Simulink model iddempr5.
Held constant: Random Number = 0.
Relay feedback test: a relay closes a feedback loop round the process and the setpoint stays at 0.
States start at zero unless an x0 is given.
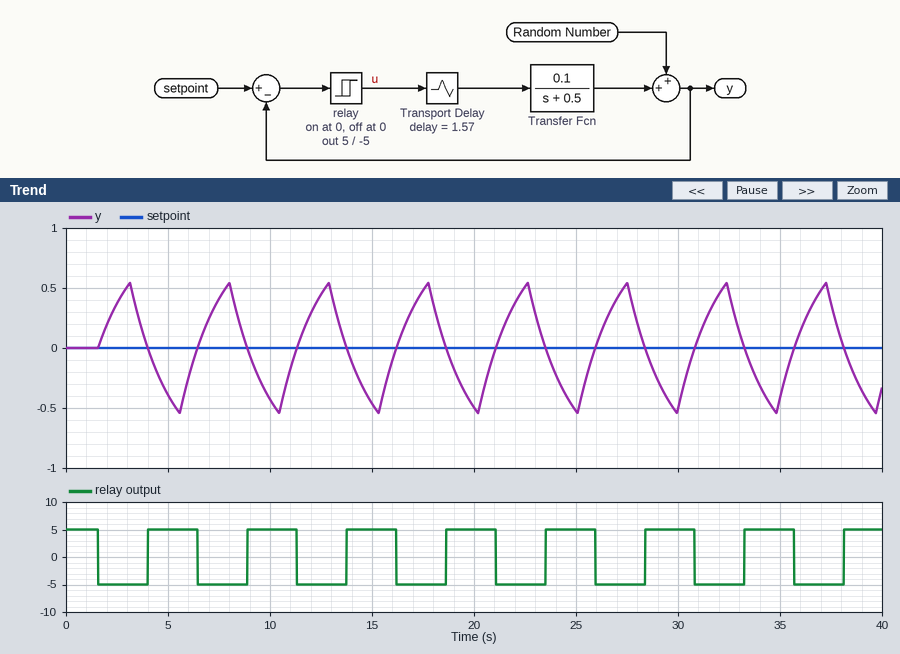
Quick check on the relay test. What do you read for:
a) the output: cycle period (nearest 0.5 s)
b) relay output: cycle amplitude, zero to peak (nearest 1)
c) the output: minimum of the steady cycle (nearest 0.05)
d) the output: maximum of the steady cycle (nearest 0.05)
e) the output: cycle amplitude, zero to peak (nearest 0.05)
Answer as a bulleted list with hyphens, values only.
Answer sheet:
- 5.0 s
- 5
- -0.55
- 0.55
- 0.55
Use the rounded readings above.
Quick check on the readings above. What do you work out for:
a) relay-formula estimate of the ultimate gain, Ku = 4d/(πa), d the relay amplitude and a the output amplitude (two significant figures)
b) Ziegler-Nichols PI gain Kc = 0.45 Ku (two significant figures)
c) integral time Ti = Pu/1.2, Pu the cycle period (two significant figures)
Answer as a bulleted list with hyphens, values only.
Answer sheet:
- 12
- 5.4
- 4.2 s
